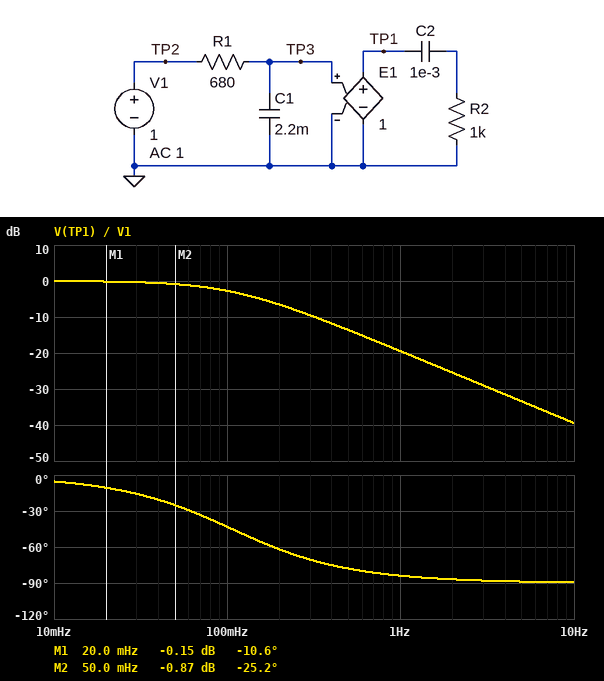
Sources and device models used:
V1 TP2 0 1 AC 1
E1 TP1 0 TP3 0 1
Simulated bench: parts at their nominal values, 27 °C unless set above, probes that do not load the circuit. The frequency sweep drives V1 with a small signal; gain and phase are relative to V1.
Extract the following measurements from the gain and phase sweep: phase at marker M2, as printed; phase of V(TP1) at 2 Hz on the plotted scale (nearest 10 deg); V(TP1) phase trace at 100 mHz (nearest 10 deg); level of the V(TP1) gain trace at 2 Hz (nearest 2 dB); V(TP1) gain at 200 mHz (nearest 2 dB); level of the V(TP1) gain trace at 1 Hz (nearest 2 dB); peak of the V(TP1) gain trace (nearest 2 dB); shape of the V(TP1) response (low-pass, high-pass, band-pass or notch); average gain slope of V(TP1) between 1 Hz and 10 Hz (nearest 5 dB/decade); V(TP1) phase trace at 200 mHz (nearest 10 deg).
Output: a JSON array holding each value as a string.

["-25.2 deg", "-90 deg", "-40 deg", "-26 dB", "-6 dB", "-20 dB", "0 dB", "low-pass", "-20 dB/decade", "-60 deg"]
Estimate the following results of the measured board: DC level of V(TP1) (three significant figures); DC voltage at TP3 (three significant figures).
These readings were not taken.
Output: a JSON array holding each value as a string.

["1.00 V", "1.00 V"]
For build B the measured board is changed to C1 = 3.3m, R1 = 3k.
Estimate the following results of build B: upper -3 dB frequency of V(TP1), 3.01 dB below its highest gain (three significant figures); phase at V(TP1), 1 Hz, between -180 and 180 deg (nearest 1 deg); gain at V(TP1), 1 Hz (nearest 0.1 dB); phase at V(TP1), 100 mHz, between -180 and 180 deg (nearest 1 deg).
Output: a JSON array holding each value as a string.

["16.1 mHz", "-89 deg", "-35.9 dB", "-81 deg"]
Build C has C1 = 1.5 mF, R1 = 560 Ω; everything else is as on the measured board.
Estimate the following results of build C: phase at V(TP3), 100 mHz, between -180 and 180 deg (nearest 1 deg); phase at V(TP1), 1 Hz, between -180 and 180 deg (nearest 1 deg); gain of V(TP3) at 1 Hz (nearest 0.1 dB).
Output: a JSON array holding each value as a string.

["-28 deg", "-79 deg", "-14.6 dB"]
